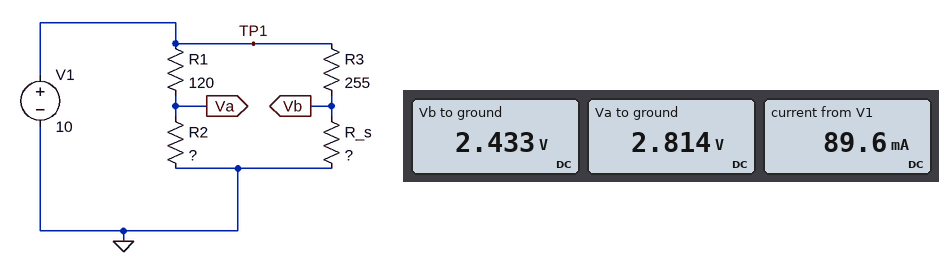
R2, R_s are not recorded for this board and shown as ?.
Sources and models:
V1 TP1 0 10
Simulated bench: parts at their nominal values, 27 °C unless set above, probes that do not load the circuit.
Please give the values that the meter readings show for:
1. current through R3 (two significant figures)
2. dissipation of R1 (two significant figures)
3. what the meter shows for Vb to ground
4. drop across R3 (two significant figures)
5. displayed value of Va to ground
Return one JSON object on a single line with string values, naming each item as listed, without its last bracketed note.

{"current through R3": "30 mA", "dissipation of R1": "430 mW", "what the meter shows for Vb to ground": "2.433 V", "drop across R3": "7.6 V", "displayed value of Va to ground": "2.814 V"}
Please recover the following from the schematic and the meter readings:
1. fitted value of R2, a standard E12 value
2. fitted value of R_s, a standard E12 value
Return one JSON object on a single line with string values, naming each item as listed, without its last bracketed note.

{"fitted value of R2, a standard E12 value": "47 Ω", "fitted value of R_s, a standard E12 value": "82 Ω"}
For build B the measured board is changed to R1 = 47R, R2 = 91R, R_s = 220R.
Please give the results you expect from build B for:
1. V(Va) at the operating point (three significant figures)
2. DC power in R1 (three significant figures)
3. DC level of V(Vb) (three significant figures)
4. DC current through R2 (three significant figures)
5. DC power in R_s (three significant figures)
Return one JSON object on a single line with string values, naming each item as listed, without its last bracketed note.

{"V(Va) at the operating point": "6.59 V", "DC power in R1": "247 mW", "DC level of V(Vb)": "4.63 V", "DC current through R2": "72.5 mA", "DC power in R_s": "97.5 mW"}
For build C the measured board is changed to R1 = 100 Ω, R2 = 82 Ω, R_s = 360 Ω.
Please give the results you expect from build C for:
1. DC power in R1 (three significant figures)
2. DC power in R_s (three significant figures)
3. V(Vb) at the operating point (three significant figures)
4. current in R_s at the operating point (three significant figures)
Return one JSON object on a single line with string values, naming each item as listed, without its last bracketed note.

{"DC power in R1": "302 mW", "DC power in R_s": "95.2 mW", "V(Vb) at the operating point": "5.85 V", "current in R_s at the operating point": "16.3 mA"}
